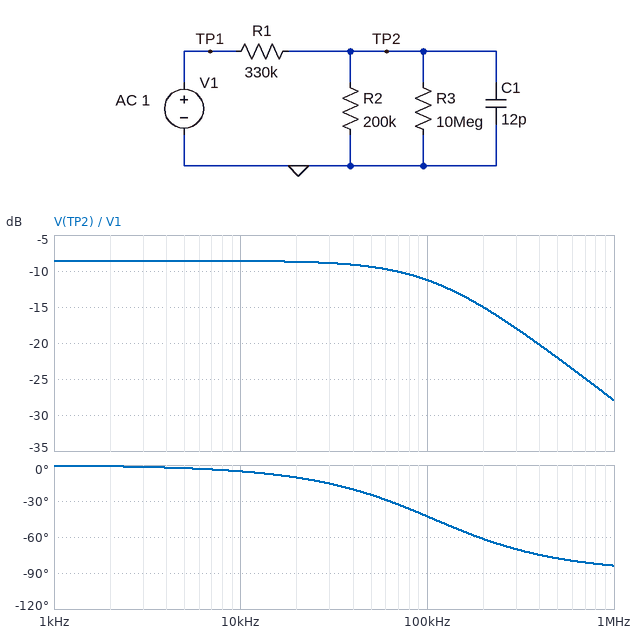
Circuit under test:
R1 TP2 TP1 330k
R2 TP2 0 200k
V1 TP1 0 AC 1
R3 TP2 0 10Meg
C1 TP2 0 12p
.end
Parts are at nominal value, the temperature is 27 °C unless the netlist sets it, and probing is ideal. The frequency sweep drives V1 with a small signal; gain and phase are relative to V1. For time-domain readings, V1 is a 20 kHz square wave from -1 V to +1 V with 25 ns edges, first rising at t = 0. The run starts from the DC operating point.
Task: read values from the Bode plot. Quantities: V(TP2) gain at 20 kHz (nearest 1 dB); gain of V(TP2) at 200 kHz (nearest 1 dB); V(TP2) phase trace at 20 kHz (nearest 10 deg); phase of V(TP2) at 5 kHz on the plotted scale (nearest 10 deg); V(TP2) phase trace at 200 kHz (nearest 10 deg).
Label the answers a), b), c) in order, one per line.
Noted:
a) -9 dB
b) -15 dB
c) -10 deg
d) 0 deg
e) -60 deg
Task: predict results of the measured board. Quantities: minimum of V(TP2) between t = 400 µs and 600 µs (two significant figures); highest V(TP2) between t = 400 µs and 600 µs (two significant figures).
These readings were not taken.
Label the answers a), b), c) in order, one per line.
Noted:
a) -370 mV
b) 370 mV
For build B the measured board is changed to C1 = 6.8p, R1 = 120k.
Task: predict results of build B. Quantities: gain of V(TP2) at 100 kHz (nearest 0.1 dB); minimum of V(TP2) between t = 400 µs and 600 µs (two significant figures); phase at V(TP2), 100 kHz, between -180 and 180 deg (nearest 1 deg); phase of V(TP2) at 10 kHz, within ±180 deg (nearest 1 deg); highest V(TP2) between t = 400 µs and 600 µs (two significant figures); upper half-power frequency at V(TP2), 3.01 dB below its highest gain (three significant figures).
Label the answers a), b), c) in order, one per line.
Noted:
a) -4.6 dB
b) -620 mV
c) -18 deg
d) -2 deg
e) 620 mV
f) 314 kHz
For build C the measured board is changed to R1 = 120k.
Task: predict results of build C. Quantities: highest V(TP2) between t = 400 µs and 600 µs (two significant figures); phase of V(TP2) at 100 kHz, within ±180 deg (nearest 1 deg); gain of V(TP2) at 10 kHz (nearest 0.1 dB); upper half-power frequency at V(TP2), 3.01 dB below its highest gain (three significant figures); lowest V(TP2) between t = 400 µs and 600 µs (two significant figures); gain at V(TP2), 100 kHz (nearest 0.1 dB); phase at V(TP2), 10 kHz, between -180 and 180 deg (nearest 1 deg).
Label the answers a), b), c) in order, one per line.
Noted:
a) 620 mV
b) -29 deg
c) -4.2 dB
d) 178 kHz
e) -620 mV
f) -5.3 dB
g) -3 deg
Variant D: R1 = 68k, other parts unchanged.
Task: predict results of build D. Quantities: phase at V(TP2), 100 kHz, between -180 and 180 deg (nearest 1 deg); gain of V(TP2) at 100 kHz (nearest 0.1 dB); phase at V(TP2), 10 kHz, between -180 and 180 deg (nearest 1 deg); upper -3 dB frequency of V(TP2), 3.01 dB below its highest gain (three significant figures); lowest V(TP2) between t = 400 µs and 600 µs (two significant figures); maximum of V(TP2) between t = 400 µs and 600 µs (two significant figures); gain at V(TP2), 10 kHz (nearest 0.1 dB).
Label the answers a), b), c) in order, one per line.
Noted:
a) -21 deg
b) -3.2 dB
c) -2 deg
d) 263 kHz
e) -740 mV
f) 740 mV
g) -2.6 dB
